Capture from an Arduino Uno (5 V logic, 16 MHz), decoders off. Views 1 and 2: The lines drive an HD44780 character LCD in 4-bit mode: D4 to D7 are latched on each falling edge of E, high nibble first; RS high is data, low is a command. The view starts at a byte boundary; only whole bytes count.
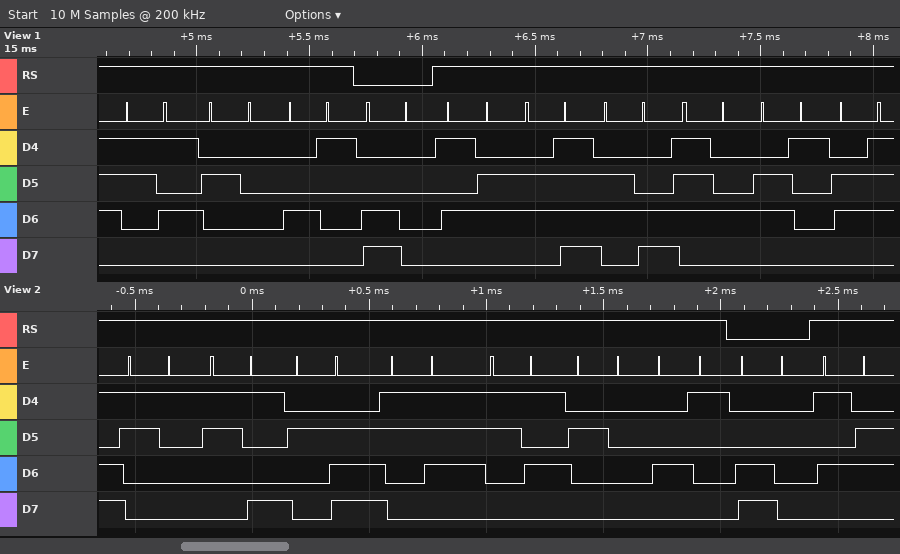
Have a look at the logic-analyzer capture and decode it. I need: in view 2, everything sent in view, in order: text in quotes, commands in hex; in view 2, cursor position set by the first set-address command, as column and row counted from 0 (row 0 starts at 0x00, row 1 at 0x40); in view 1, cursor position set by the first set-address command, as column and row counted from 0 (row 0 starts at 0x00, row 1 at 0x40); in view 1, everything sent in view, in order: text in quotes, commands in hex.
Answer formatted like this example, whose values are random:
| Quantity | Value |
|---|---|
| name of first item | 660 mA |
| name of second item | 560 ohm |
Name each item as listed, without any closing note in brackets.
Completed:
| Quantity | Value |
|---|---|
| in view 2, everything sent in view, in order: text in quotes, commands in hex | "19.75 A" 0xC0 "V" |
| in view 2, cursor position set by the first set-address command, as column and row counted from 0 | column 0, row 1 |
| in view 1, cursor position set by the first set-address command, as column and row counted from 0 | column 0, row 1 |
| in view 1, everything sent in view, in order: text in quotes, commands in hex | "5 A" 0xC0 "Voltag" |
